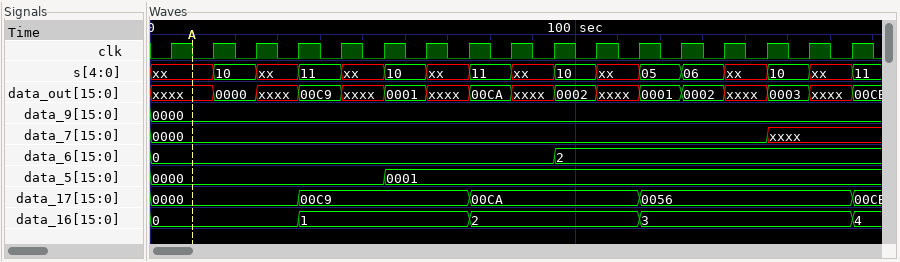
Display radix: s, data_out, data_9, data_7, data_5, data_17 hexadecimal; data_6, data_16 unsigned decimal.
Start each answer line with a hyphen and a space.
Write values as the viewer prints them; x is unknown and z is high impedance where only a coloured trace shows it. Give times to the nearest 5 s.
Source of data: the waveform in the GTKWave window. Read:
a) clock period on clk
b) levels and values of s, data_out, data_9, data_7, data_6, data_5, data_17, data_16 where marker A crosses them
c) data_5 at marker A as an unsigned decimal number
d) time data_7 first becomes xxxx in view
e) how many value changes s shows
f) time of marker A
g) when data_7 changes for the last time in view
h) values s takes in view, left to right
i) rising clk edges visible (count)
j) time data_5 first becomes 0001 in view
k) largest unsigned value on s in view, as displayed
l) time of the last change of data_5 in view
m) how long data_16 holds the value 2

- 10 s
- s=xx, data_out=xxxx, data_9=0000, data_7=0000, data_6=0, data_5=0000, data_17=0000, data_16=0
- 0
- 145 s
- 16
- 10 s
- 145 s
- xx, 10, xx, 11, xx, 10, xx, 11, xx, 10, xx, 05, 06, xx, 10, xx, 11
- 17
- 55 s
- 11
- 55 s
- 40 s
